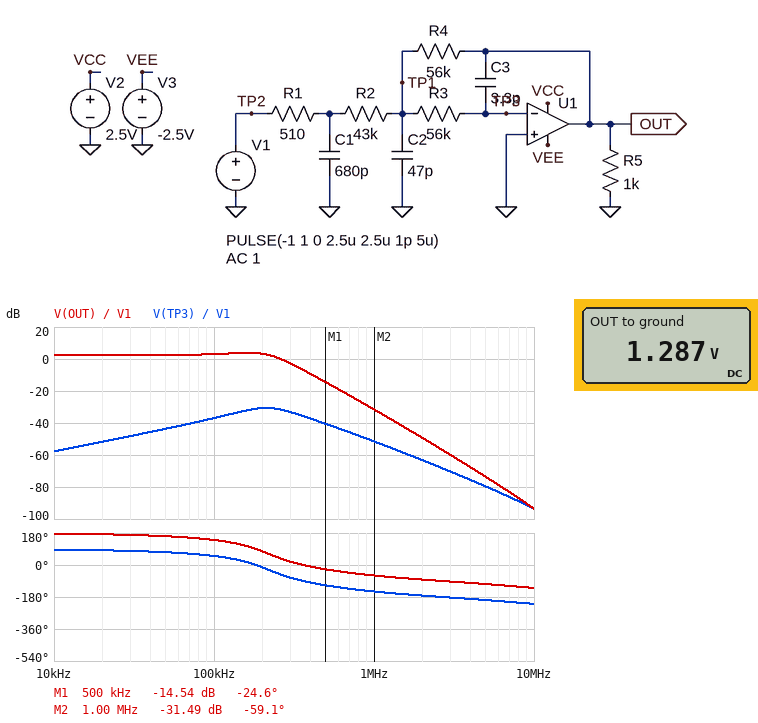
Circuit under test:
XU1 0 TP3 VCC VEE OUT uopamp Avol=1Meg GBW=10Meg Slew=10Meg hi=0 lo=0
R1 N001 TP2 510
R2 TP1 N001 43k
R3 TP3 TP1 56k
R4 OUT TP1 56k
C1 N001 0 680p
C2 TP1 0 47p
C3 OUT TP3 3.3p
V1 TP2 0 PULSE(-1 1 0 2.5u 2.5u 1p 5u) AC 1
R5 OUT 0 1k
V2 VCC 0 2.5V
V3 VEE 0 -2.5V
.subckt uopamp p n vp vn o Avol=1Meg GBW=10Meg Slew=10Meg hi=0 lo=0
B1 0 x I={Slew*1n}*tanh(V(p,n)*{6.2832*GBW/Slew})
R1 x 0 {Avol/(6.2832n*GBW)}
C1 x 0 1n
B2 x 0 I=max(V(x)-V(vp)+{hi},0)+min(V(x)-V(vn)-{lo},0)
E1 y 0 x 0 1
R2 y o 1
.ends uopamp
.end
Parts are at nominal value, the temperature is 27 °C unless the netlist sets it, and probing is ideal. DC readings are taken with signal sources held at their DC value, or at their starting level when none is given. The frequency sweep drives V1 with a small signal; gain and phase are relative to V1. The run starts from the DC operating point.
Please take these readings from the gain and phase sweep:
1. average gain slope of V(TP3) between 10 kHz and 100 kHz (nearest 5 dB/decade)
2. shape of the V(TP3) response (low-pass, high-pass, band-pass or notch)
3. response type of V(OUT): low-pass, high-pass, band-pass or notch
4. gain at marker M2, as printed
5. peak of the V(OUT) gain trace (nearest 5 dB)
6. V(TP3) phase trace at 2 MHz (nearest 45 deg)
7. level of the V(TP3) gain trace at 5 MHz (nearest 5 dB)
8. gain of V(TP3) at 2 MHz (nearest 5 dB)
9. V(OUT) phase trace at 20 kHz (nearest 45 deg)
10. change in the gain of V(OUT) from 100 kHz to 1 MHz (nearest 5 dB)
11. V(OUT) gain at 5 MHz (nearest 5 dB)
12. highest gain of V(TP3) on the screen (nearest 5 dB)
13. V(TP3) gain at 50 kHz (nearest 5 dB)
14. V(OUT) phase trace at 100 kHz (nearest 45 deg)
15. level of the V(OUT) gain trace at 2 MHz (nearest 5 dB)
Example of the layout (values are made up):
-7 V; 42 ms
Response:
20 dB/decade; band-pass; low-pass; -31.49 dB; 5 dB; -180 deg; -80 dB; -65 dB; 180 deg; -35 dB; -75 dB; -30 dB; -45 dB; 135 deg; -50 dB
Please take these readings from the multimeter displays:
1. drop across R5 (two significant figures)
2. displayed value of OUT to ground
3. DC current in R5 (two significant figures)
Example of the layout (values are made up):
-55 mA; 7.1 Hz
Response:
1.3 V; 1.287 V; 1.3 mA
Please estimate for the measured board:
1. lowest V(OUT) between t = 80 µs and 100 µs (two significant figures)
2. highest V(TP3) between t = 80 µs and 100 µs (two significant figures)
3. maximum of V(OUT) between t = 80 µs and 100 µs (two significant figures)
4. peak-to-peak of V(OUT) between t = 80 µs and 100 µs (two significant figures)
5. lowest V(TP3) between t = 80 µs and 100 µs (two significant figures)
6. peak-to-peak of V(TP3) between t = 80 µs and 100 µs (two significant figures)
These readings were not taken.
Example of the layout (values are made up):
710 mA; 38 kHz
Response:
-1.2 V; 24 mV; 1.2 V; 2.4 V; -24 mV; 48 mV
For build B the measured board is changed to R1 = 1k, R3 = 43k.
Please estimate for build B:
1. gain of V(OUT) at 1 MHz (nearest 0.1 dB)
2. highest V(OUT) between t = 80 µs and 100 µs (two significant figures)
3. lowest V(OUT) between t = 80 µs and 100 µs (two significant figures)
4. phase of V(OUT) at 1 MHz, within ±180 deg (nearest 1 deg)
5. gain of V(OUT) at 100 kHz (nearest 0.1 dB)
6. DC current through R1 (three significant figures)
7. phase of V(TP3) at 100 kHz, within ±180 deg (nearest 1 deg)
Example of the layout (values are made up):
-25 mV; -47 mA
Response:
-34.6 dB; 1.1 V; -1.1 V; -69 deg; 2.3 dB; 22.7 µA; 45 deg
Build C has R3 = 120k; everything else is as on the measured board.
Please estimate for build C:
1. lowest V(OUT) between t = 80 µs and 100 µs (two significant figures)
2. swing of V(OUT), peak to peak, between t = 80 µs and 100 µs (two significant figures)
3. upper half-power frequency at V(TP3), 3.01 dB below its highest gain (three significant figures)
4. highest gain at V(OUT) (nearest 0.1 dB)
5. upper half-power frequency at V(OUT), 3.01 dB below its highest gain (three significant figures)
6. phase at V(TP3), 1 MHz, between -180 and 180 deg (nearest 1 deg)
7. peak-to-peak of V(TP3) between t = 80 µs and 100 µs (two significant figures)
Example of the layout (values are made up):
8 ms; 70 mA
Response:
-610 mV; 1.2 V; 239 kHz; 2.9 dB; 171 kHz; -151 deg; 25 mV
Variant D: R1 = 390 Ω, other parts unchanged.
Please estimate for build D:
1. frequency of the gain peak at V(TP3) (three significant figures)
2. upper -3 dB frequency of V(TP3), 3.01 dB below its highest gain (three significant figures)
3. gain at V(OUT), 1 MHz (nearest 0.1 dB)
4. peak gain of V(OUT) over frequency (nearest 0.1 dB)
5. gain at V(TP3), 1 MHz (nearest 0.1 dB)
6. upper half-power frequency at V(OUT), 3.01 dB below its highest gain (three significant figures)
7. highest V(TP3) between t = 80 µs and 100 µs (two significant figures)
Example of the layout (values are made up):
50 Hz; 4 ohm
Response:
214 kHz; 317 kHz; -29.7 dB; 4.0 dB; -49.7 dB; 253 kHz; 25 mV
